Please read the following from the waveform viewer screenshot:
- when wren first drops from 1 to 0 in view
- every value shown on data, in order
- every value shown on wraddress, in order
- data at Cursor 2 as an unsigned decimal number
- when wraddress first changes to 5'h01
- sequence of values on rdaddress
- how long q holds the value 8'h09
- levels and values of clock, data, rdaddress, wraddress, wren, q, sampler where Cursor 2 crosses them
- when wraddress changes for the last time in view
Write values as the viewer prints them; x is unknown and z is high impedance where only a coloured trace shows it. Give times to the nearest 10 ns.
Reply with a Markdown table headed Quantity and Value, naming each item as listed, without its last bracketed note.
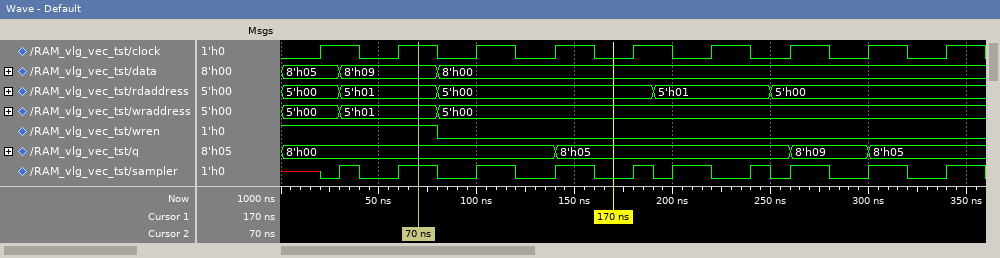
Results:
| Quantity | Value |
|---|---|
| when wren first drops from 1 to 0 in view | 80 ns |
| every value shown on data, in order | 8'h05, 8'h09, 8'h00 |
| every value shown on wraddress, in order | 5'h00, 5'h01, 5'h00 |
| data at Cursor 2 as an unsigned decimal number | 9 |
| when wraddress first changes to 5'h01 | 30 ns |
| sequence of values on rdaddress | 5'h00, 5'h01, 5'h00, 5'h01, 5'h00 |
| how long q holds the value 8'h09 | 40 ns |
| levels and values of clock, data, rdaddress, wraddress, wren, q, sampler where Cursor 2 crosses them | clock=1, data=8'h09, rdaddress=5'h01, wraddress=5'h01, wren=1, q=8'h00, sampler=1 |
| when wraddress changes for the last time in view | 80 ns |
